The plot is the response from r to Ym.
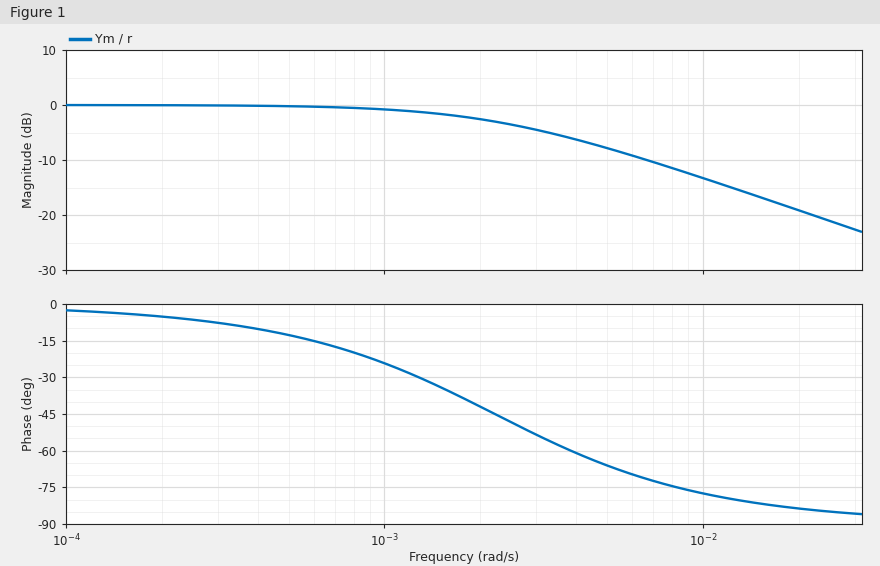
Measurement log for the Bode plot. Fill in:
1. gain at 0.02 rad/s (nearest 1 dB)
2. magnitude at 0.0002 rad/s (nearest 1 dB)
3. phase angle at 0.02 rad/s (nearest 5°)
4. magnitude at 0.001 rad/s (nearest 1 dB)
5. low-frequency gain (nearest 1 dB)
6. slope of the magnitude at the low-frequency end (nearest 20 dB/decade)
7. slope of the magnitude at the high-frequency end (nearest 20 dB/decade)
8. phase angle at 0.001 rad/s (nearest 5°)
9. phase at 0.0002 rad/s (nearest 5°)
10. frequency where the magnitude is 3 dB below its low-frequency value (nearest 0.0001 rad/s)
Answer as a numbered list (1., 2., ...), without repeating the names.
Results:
1. -19 dB
2. 0 dB
3. -85°
4. -1 dB
5. 0 dB
6. 0 dB/decade
7. -20 dB/decade
8. -25°
9. -5°
10. 0.0022 rad/s
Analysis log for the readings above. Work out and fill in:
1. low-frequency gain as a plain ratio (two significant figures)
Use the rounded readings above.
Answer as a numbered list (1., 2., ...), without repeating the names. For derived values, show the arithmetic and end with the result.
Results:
1. 10^(0 / 20) = 1.0
